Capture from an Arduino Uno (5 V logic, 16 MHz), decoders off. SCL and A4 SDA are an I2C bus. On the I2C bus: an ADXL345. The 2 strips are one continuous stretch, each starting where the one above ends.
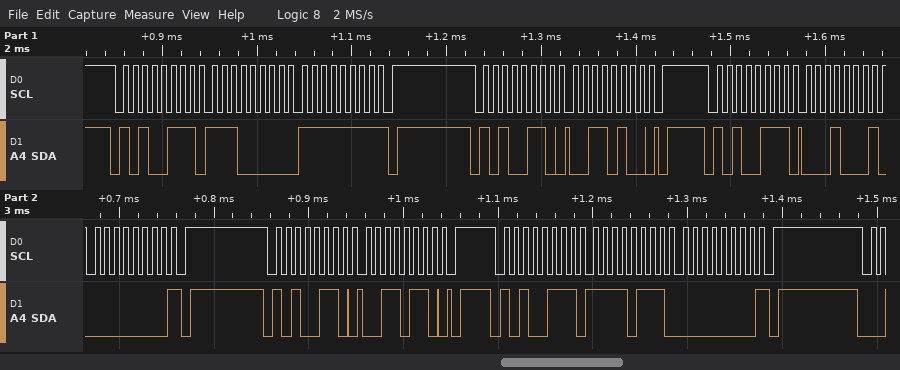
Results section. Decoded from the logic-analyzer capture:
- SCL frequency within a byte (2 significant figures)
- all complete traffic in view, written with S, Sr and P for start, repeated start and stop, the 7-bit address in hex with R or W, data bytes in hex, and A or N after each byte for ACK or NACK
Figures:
100 kHz
S 53R A E0 A FF N P S 53W A 34 A P S 53R A 11 A 00 N P S 53W A 36 A P S 53R A F7 A 00 N P
